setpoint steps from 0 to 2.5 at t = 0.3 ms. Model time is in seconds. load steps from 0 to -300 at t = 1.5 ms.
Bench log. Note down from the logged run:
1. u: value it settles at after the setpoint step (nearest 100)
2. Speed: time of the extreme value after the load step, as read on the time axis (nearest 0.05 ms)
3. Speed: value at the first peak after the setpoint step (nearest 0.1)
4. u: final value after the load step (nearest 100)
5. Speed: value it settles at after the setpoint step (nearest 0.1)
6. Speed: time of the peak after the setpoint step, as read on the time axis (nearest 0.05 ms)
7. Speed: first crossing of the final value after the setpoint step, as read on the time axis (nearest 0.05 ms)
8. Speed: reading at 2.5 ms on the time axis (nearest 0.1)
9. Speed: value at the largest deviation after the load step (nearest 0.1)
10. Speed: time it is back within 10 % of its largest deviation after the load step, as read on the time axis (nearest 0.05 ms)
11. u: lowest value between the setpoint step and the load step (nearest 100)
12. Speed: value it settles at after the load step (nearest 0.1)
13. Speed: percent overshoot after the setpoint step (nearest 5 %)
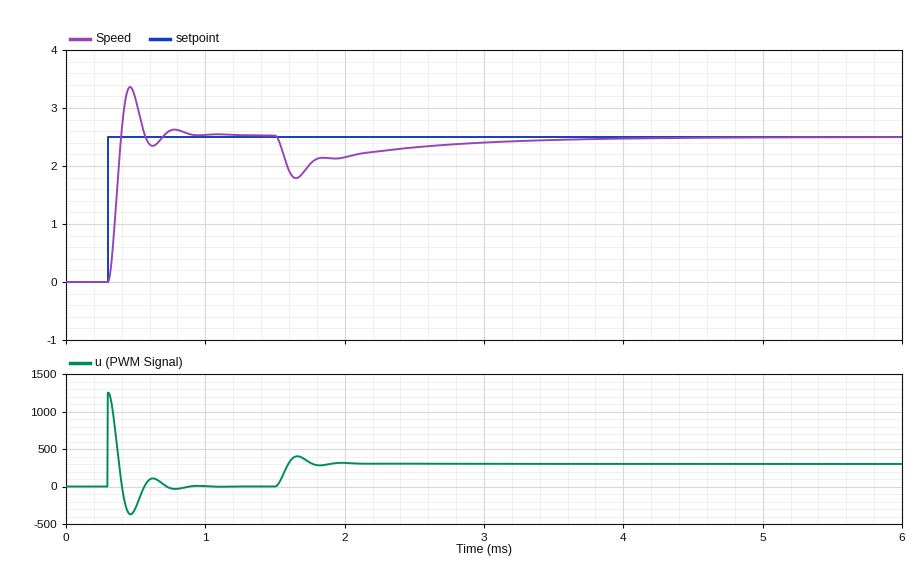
0
1.65 ms
3.4
300
2.5
0.45 ms
0.40 ms
2.3
1.8
3.20 ms
-400
2.5
35 %
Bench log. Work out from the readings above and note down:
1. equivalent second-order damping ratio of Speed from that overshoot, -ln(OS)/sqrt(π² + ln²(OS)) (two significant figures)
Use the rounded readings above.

0.32
